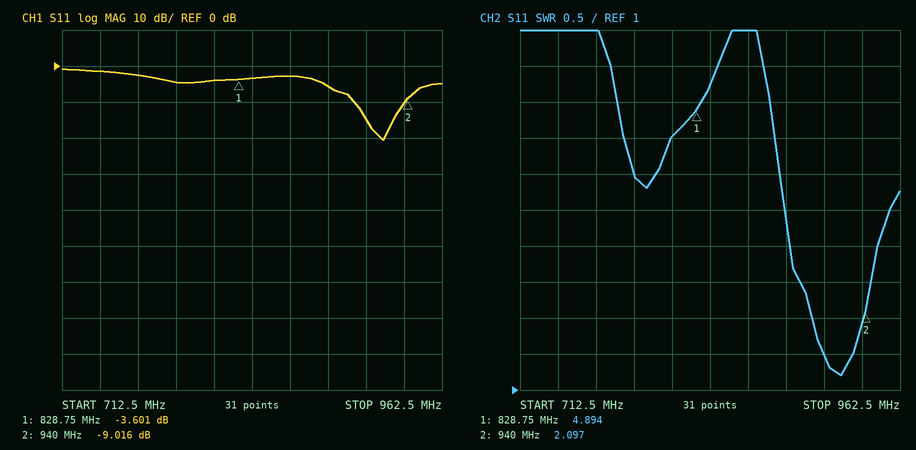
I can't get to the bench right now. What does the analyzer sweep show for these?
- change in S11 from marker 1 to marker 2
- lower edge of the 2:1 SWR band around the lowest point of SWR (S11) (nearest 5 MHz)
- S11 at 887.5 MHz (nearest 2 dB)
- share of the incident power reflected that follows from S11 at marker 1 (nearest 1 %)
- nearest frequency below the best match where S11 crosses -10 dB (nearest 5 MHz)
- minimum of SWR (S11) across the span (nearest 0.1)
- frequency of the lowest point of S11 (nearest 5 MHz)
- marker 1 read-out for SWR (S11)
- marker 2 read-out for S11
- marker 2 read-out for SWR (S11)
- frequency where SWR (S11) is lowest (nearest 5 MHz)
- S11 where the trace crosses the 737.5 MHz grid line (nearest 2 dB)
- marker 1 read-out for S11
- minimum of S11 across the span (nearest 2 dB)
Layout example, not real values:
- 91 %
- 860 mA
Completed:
- -5.415 dB
- 905 MHz
- -6 dB
- 44 %
- 905 MHz
- 1.2
- 925 MHz
- 4.894
- -9.016 dB
- 2.097
- 925 MHz
- -2 dB
- -3.601 dB
- -20 dB
